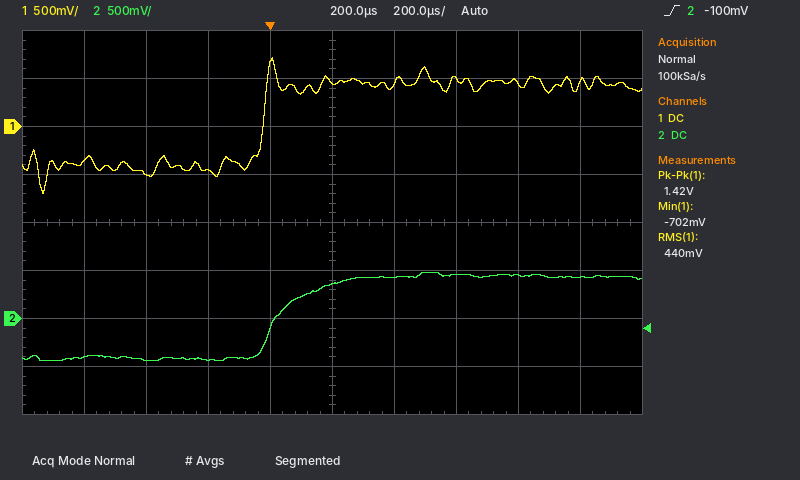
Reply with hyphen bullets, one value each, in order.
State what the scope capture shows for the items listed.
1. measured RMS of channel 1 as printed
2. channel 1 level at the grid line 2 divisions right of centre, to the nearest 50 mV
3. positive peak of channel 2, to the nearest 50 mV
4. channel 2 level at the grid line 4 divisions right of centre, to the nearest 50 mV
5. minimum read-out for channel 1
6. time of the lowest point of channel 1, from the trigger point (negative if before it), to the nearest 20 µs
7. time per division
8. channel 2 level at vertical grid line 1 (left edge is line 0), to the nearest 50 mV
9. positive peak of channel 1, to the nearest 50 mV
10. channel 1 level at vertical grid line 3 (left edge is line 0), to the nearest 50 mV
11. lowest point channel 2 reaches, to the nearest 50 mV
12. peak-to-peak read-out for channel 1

- 440 mV
- 500 mV
- 500 mV
- 450 mV
- -702 mV
- -740 µs
- 200 µs
- -400 mV
- 700 mV
- -450 mV
- -450 mV
- 1.42 V
